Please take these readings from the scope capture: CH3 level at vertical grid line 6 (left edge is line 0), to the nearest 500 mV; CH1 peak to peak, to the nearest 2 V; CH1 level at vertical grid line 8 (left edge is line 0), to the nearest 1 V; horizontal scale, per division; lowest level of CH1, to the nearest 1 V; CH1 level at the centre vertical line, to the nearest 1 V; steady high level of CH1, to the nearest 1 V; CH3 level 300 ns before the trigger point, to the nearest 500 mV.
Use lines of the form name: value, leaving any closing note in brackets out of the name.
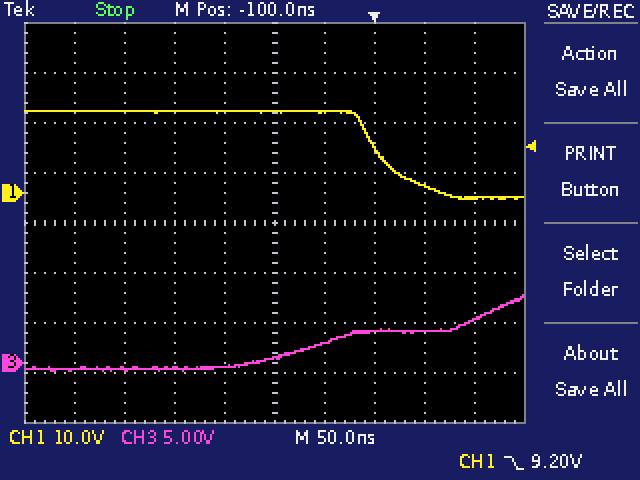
CH3 level at vertical grid line 6 (left edge is line 0), to the nearest 500 mV: 2.0 V
CH1 peak to peak, to the nearest 2 V: 18 V
CH1 level at vertical grid line 8 (left edge is line 0), to the nearest 1 V: 1 V
horizontal scale, per division: 50 ns
lowest level of CH1, to the nearest 1 V: -1 V
CH1 level at the centre vertical line, to the nearest 1 V: 16 V
steady high level of CH1, to the nearest 1 V: 16 V
CH3 level 300 ns before the trigger point, to the nearest 500 mV: -500 mV
